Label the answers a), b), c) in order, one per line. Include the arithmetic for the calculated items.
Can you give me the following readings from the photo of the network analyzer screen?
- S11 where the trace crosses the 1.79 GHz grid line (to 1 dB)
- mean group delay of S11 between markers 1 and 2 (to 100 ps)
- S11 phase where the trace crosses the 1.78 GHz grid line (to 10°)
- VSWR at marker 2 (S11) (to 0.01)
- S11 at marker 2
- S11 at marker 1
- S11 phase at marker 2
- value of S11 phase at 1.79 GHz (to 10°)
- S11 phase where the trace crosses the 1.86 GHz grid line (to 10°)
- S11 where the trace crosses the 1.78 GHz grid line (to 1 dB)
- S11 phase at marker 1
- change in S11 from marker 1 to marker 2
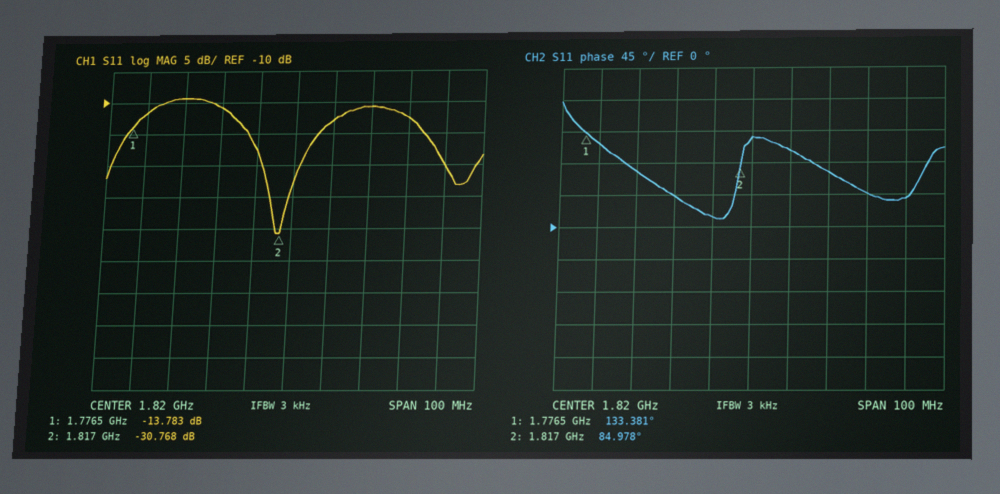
a) -9 dB
b) −(84.978° − (133.381°))/(360° × 40.5 MHz) ≈ 3.3 ns
c) 120°
d) (1 + 0.0289)/(1 − 0.0289) ≈ 1.06
e) -30.768 dB
f) -13.783 dB
g) 84.978°
h) 80°
i) 40°
j) -12 dB
k) 133.381°
l) -30.768 − (-13.783) = -16.985 dB
